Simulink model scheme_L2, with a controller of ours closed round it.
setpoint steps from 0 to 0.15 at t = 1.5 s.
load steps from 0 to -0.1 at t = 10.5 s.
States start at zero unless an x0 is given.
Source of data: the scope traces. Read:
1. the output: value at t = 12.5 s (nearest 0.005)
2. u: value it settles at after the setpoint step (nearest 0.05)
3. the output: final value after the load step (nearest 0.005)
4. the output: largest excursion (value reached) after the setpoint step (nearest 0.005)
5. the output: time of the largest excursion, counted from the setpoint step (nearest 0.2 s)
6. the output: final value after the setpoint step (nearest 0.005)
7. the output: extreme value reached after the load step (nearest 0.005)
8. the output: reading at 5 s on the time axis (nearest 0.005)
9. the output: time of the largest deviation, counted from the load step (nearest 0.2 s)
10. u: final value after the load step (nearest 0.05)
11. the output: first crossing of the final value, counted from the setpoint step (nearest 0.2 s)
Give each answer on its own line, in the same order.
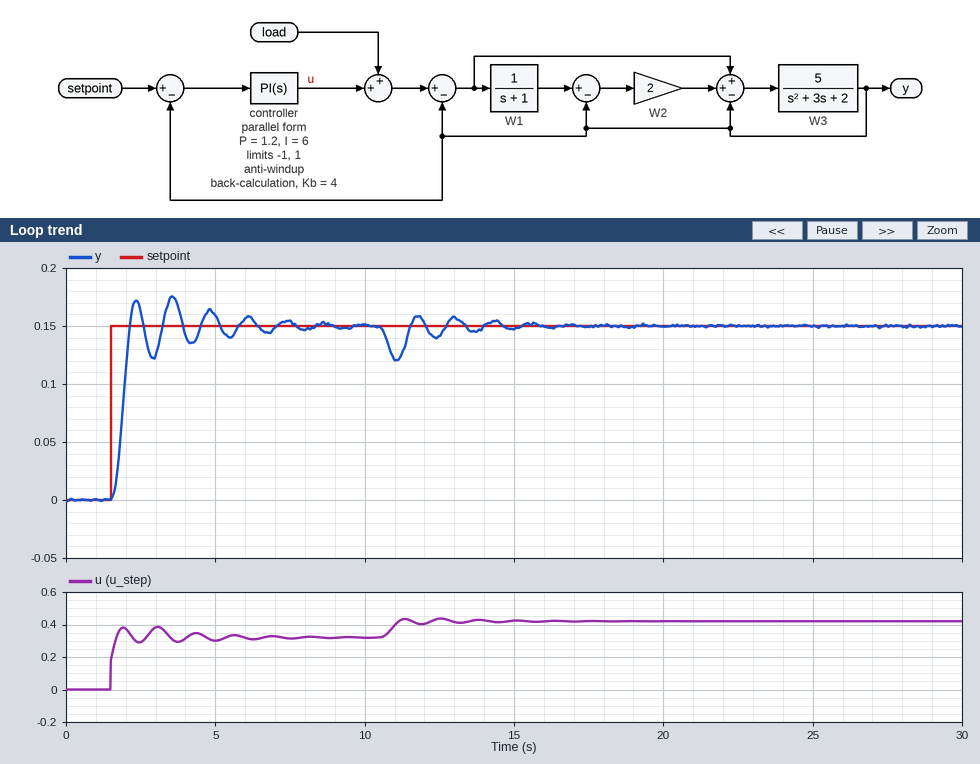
0.140
0.30
0.150
0.175
2.0 s
0.150
0.120
0.160
0.6 s
0.40
0.6 s
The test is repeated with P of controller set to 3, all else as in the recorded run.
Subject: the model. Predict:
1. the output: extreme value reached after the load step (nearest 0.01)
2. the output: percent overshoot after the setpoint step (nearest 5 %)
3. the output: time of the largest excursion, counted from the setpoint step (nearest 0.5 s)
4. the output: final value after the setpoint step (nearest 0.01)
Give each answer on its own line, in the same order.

0.13
20 %
1.5 s
0.15
